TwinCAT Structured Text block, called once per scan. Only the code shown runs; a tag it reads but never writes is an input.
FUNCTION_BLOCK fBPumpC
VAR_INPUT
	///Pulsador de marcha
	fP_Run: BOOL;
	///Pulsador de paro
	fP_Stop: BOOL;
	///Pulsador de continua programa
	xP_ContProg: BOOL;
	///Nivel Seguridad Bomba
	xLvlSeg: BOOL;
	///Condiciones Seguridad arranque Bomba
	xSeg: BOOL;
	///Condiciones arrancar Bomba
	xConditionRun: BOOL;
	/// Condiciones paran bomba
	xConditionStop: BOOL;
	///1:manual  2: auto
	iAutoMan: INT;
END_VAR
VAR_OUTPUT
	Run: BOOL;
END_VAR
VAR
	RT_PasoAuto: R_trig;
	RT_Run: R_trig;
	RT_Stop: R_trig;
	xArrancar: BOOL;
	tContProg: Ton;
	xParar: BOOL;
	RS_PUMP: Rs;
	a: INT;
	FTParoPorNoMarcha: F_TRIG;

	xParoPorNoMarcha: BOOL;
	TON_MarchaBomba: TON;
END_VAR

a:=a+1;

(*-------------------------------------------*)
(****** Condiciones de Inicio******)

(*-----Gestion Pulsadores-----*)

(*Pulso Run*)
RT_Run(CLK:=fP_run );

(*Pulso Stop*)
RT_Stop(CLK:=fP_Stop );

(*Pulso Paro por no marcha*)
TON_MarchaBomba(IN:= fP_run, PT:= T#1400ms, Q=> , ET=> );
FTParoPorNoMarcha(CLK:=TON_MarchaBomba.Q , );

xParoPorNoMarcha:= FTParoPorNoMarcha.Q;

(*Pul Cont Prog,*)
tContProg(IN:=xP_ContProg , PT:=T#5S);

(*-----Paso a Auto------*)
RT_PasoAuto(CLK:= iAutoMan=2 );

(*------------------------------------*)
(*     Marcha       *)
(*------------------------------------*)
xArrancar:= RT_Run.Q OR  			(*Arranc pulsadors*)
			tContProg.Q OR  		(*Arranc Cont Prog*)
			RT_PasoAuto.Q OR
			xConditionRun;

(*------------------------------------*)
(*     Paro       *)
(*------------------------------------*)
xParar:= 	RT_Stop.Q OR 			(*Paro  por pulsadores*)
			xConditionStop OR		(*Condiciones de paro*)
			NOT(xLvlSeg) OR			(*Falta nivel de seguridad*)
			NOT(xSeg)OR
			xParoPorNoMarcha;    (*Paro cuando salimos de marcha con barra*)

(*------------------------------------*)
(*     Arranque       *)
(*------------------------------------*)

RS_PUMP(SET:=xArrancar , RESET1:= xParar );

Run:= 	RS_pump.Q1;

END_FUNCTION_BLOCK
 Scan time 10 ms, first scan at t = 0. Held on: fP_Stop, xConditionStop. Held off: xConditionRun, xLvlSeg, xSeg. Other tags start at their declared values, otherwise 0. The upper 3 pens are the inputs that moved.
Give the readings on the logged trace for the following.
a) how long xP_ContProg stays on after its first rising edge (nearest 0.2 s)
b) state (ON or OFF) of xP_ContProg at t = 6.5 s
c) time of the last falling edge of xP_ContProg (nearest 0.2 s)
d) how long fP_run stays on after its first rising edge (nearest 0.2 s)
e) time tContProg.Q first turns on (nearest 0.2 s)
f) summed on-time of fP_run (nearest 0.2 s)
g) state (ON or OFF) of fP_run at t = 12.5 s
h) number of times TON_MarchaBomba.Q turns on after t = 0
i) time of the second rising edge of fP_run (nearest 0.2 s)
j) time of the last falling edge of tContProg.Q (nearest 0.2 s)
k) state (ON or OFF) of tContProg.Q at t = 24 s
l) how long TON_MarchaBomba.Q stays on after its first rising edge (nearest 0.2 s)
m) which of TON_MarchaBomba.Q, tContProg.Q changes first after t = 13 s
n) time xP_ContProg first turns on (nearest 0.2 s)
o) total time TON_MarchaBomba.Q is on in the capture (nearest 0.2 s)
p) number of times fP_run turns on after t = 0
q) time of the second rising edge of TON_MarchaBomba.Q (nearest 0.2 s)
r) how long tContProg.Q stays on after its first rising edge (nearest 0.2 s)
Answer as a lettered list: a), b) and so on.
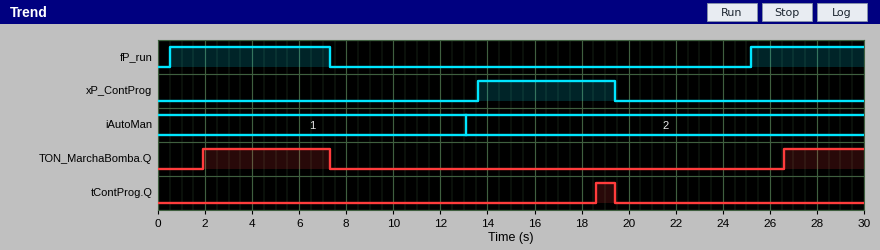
a) 5.8 s
b) OFF
c) 19.4 s
d) 6.8 s
e) 18.6 s
f) 11.6 s
g) OFF
h) 2
i) 25.2 s
j) 19.4 s
k) OFF
l) 5.4 s
m) tContProg.Q
n) 13.6 s
o) 8.8 s
p) 2
q) 26.6 s
r) 0.8 s
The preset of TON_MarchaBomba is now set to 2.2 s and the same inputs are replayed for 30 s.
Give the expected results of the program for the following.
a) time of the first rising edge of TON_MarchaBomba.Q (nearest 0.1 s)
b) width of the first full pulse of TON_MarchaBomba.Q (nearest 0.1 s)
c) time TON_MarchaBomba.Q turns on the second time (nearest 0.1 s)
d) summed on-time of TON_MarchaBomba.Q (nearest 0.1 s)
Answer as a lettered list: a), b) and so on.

a) 2.7 s
b) 4.6 s
c) 27.4 s
d) 7.2 s
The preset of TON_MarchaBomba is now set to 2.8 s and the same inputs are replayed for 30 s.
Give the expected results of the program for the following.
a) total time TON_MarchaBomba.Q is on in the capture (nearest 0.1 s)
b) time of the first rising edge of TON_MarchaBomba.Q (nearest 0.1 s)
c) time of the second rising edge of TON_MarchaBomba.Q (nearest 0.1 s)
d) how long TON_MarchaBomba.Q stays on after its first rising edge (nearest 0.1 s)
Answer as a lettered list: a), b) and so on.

a) 6.0 s
b) 3.3 s
c) 28.0 s
d) 4.0 s
